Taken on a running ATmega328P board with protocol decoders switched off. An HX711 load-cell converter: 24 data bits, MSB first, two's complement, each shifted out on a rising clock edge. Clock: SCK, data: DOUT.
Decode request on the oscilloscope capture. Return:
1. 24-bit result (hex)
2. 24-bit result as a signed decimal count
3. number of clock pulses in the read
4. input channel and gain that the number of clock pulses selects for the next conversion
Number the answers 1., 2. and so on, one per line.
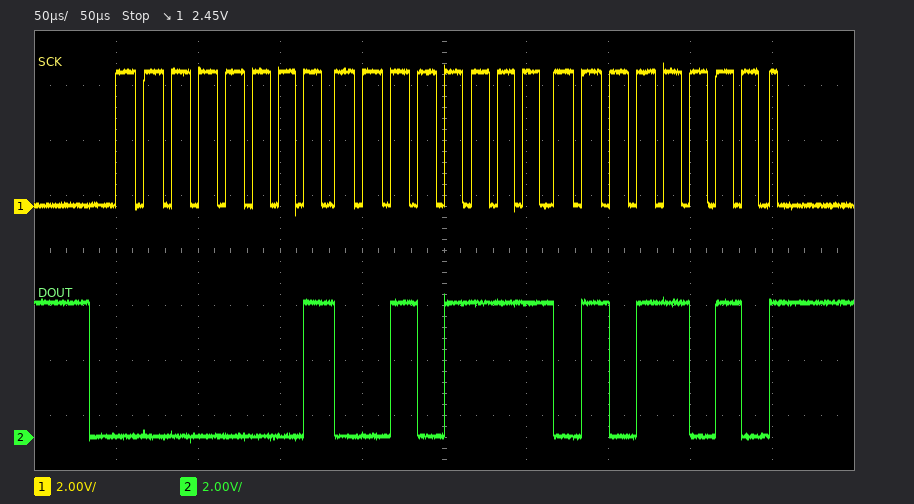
1. 0x012F5A
2. 77658
3. 25
4. channel A, gain 128
